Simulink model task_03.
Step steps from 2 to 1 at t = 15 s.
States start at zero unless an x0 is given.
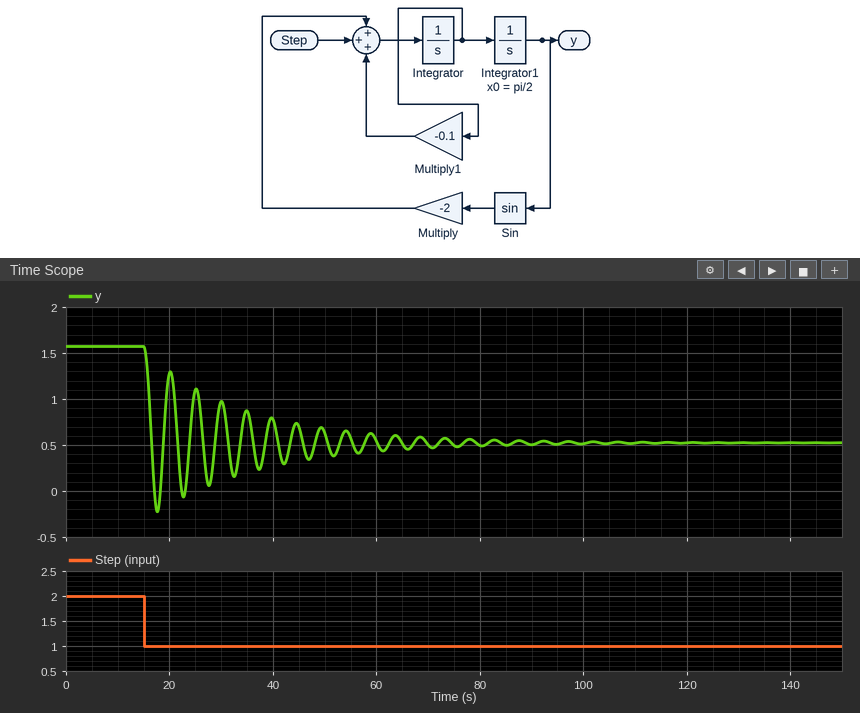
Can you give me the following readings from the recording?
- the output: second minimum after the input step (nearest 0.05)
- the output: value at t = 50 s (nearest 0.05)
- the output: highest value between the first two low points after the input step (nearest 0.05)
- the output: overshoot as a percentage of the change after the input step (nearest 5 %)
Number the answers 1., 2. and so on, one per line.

1. -0.05
2. 0.65
3. 1.30
4. 70 %
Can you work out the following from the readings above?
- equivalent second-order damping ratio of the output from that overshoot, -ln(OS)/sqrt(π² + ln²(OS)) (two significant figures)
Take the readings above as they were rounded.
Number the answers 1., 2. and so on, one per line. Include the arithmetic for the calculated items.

1. ln(0.7) = -0.357; 0.357 / sqrt(9.870 + 0.127) = 0.11
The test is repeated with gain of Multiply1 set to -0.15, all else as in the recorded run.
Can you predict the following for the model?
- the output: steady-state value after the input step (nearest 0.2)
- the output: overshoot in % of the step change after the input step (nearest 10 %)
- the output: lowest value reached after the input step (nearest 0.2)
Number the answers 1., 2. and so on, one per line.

1. 0.6
2. 70 %
3. -0.2
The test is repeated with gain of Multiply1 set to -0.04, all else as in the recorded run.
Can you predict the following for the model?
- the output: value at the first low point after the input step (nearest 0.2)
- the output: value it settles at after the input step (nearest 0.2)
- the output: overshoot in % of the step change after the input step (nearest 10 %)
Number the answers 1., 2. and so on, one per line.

1. -0.2
2. 0.6
3. 80 %
